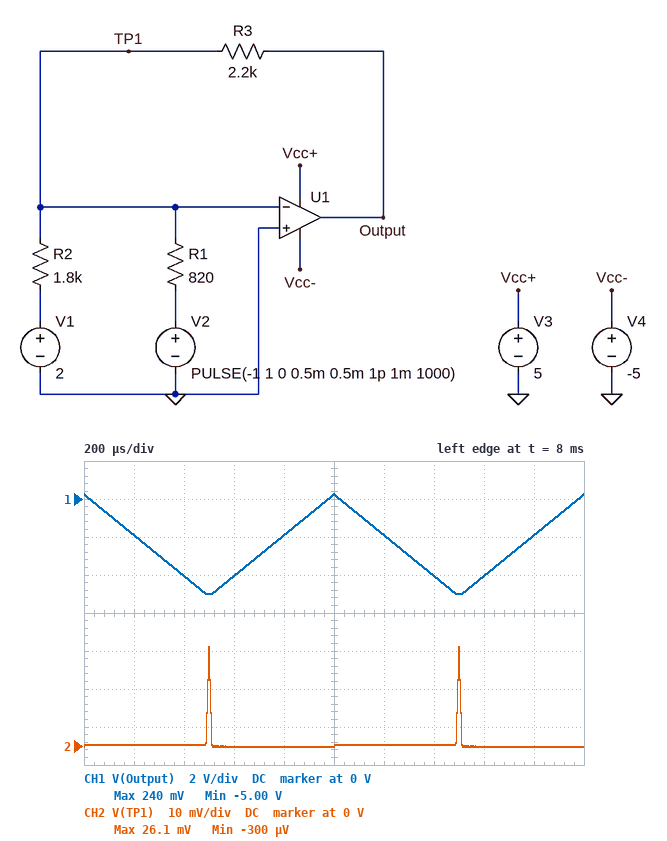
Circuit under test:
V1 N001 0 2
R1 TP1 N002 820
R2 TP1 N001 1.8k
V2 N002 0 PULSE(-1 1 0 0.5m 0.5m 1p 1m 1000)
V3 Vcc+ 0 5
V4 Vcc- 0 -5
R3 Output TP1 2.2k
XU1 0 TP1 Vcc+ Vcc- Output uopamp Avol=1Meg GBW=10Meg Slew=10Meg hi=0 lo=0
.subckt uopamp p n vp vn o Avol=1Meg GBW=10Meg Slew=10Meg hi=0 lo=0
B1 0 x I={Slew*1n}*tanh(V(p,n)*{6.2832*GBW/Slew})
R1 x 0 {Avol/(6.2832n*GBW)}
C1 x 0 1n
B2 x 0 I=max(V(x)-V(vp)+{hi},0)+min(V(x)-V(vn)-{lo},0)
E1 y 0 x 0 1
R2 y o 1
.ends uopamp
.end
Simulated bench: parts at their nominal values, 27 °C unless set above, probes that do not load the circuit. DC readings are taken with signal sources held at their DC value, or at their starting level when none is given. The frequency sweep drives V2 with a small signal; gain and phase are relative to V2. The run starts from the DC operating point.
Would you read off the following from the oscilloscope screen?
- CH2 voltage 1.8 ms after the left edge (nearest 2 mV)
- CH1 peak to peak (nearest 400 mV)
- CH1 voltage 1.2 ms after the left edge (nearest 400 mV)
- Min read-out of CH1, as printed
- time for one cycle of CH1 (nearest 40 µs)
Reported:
0 V
5.2 V
-2.0 V
-5.00 V
1.00 ms
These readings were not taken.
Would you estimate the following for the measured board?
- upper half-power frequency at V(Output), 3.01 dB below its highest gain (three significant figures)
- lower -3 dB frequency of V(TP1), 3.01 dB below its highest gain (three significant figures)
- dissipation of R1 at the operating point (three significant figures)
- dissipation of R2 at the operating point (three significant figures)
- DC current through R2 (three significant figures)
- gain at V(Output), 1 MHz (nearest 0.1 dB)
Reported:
2.04 MHz
2.04 MHz
1.22 mW
2.22 mW
1.11 mA
7.6 dB
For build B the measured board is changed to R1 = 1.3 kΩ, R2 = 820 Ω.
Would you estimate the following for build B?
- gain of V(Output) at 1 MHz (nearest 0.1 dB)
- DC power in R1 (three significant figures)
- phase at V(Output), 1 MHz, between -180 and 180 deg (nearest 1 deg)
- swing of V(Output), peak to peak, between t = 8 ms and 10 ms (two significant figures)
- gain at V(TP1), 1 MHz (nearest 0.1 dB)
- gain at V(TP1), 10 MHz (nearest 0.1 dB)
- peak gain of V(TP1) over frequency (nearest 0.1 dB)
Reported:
3.5 dB
769 µW
152 deg
1.3 V
-16.5 dB
-10.2 dB
-10.0 dB
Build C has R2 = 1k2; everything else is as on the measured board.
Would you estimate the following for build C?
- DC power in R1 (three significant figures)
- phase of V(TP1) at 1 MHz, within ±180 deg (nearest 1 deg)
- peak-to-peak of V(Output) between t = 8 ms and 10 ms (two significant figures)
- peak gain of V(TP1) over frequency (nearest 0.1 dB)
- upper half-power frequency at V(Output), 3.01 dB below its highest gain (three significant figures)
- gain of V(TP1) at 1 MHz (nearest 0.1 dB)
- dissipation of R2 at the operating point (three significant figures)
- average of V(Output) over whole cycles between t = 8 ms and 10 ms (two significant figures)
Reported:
1.22 mW
61 deg
4.0 V
-6.3 dB
1.81 MHz
-12.6 dB
3.33 mW
-3.5 V
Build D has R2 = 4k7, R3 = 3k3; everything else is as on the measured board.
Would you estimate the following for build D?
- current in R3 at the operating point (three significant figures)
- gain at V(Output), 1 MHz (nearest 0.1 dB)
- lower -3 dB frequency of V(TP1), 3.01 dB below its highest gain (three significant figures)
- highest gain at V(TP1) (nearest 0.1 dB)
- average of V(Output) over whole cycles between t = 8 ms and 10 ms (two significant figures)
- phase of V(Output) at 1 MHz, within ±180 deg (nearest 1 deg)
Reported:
794 µA
10.9 dB
1.75 MHz
-3.1 dB
-1.4 V
150 deg
